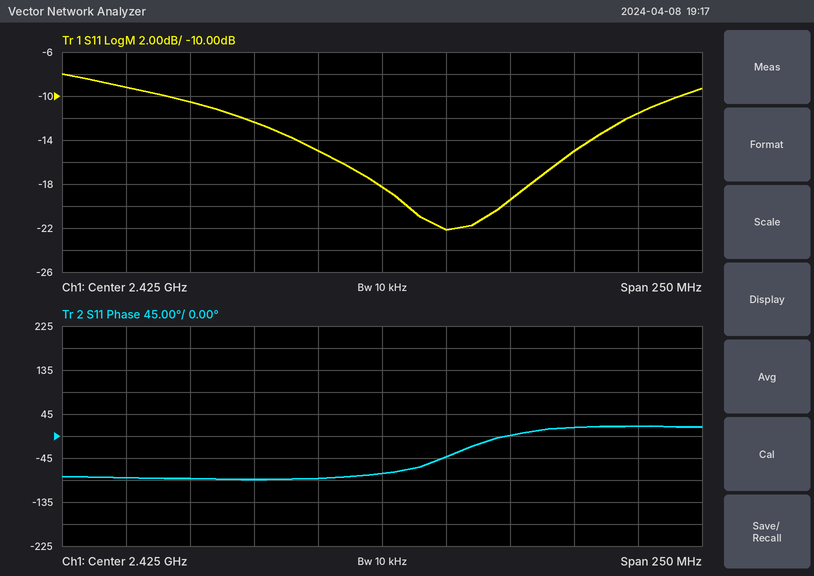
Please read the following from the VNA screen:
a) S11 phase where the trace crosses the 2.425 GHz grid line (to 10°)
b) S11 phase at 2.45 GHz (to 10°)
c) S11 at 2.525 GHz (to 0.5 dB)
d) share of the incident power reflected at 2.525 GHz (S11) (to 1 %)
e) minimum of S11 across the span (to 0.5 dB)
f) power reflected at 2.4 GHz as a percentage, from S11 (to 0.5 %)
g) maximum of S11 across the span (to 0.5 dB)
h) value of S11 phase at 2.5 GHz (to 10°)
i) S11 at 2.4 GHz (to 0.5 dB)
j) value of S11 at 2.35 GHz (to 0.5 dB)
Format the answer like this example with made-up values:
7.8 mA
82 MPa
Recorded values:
-80°
-40°
-11.5 dB
7 %
-22.0 dB
3.0 %
-8.0 dB
20°
-15.0 dB
-10.5 dB
